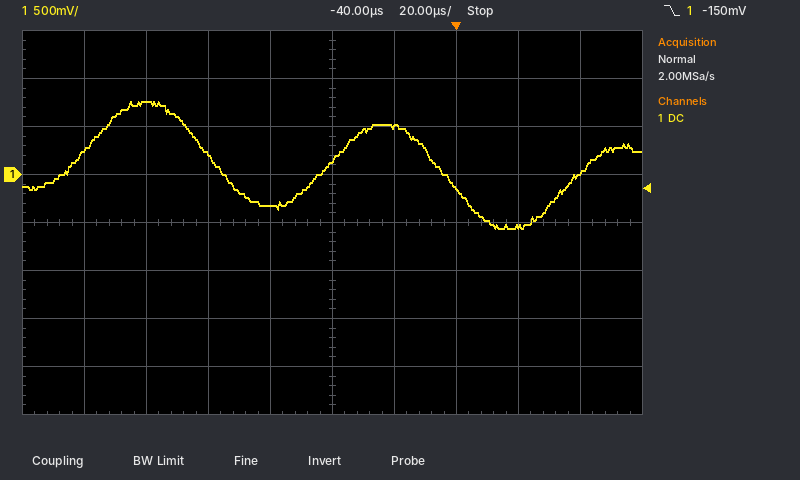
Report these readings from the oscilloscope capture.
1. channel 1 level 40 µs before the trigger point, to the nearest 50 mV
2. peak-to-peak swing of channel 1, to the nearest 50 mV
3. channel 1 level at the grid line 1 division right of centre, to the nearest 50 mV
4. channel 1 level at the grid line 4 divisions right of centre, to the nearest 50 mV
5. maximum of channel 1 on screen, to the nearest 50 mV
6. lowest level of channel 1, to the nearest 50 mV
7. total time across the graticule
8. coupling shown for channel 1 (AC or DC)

150 mV
1.30 V
500 mV
0 mV
750 mV
-550 mV
200 µs
DC
